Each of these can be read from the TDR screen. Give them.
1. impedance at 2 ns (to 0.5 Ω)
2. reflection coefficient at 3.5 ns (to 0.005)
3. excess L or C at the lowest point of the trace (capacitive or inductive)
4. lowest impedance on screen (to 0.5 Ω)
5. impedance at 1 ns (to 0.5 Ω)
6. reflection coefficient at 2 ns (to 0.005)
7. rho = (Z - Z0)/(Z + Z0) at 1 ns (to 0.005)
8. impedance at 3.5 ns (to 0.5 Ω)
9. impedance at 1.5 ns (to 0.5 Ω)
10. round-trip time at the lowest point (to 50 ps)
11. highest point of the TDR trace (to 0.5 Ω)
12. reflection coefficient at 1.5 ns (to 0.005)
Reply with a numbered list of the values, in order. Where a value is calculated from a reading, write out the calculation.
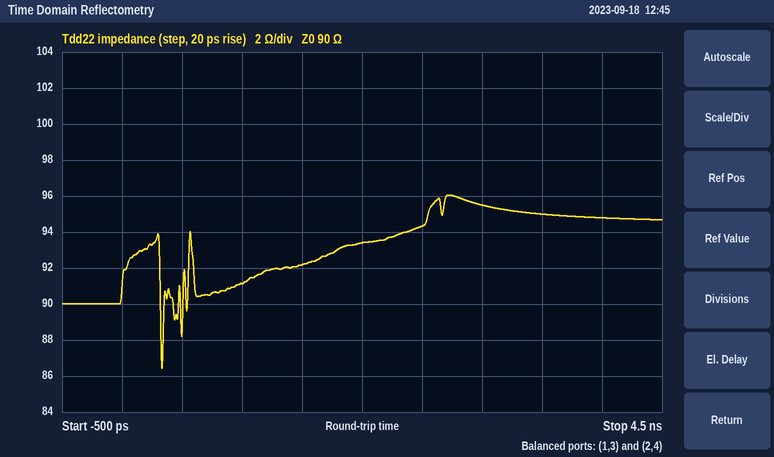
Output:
1. 93.5 Ω
2. (95 − 90)/(95 + 90) ≈ +0.0270, so +0.025 to the nearest 0.005
3. capacitive
4. 86.5 Ω
5. 91.0 Ω
6. (93.5 − 90)/(93.5 + 90) ≈ +0.0191, so +0.020 to the nearest 0.005
7. (91 − 90)/(91 + 90) ≈ +0.00552, so +0.005 to the nearest 0.005
8. 95.0 Ω
9. 92.0 Ω
10. 350 ps
11. 96.0 Ω
12. (92 − 90)/(92 + 90) ≈ +0.0110, so +0.010 to the nearest 0.005
